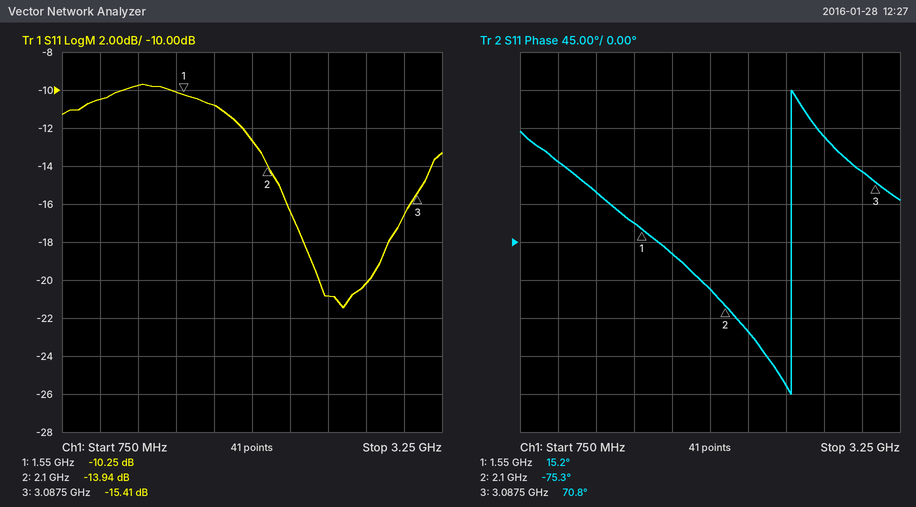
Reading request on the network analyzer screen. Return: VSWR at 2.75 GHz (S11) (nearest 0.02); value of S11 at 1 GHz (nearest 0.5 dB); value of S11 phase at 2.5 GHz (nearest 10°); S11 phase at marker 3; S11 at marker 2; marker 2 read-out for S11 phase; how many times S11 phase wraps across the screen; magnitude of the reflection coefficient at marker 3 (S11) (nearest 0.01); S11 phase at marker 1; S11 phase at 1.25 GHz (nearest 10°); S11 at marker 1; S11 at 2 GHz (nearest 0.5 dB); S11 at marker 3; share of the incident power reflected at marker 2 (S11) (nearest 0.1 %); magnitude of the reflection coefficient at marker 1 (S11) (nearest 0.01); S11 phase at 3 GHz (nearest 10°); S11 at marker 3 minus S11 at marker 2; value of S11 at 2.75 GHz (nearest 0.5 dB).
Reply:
1.22
-10.5 dB
-170°
70.8°
-13.94 dB
-75.3°
1
0.17
15.2°
60°
-10.25 dB
-12.5 dB
-15.41 dB
4.0 %
0.31
80°
-1.47 dB
-20.0 dB
